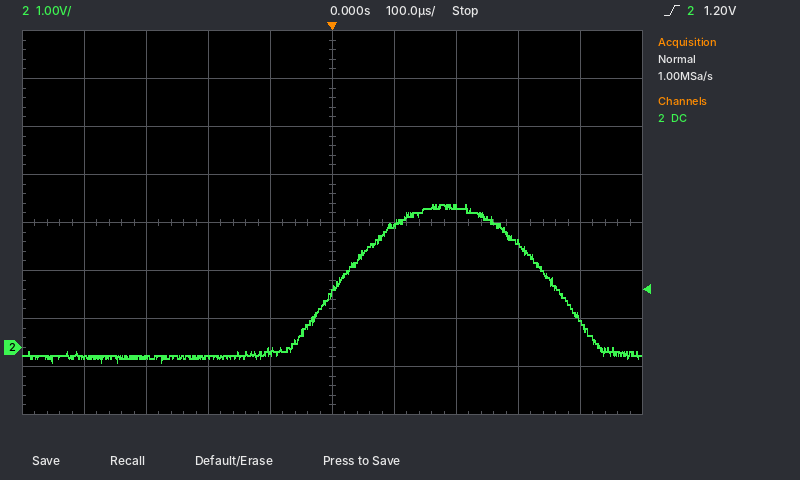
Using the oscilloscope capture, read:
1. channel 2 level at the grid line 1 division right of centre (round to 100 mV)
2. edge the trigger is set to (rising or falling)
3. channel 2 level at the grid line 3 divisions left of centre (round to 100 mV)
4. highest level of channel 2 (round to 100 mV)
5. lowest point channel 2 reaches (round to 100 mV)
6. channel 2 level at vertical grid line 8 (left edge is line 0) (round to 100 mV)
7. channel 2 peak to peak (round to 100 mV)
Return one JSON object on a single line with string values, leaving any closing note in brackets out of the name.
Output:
{"channel 2 level at the grid line 1 division right of centre": "2.6 V", "edge the trigger is set to": "rising", "channel 2 level at the grid line 3 divisions left of centre": "-200 mV", "highest level of channel 2": "3.0 V", "lowest point channel 2 reaches": "-300 mV", "channel 2 level at vertical grid line 8 (left edge is line 0)": "2.2 V", "channel 2 peak to peak": "3.3 V"}
